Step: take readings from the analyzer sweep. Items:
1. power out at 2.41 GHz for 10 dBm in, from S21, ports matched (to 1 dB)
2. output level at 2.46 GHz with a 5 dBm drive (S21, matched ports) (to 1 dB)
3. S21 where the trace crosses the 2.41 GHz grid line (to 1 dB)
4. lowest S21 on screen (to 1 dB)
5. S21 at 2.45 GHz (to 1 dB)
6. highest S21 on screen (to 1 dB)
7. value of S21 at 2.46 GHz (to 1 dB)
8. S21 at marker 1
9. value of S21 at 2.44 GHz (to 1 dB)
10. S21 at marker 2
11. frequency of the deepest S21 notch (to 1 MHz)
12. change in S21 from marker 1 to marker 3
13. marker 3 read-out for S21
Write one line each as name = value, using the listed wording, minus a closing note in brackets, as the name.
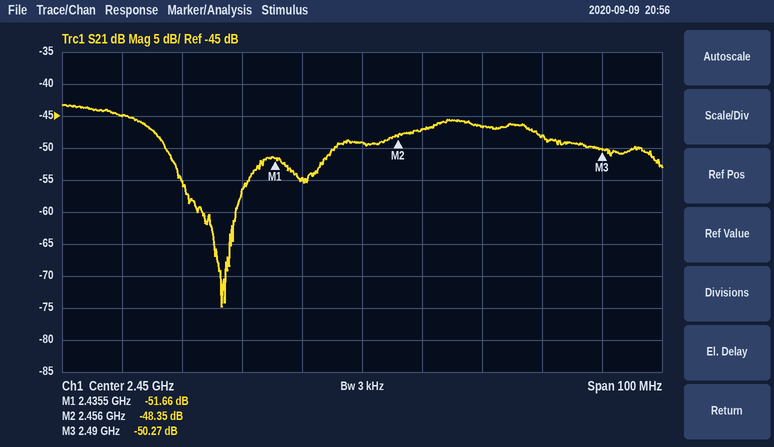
power out at 2.41 GHz for 10 dBm in, from S21, ports matched = -35 dBm
output level at 2.46 GHz with a 5 dBm drive (S21, matched ports) = -42 dBm
S21 where the trace crosses the 2.41 GHz grid line = -45 dB
lowest S21 on screen = -75 dB
S21 at 2.45 GHz = -49 dB
highest S21 on screen = -43 dB
value of S21 at 2.46 GHz = -47 dB
S21 at marker 1 = -51.66 dB
value of S21 at 2.44 GHz = -55 dB
S21 at marker 2 = -48.35 dB
frequency of the deepest S21 notch = 2.427 GHz
change in S21 from marker 1 to marker 3 = 1.39 dB
marker 3 read-out for S21 = -50.27 dB
